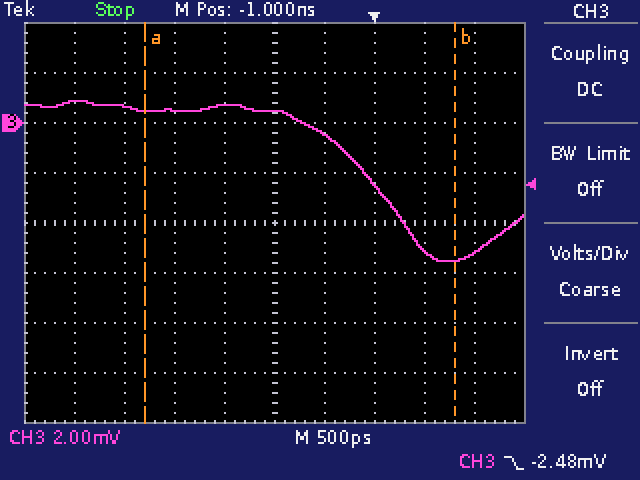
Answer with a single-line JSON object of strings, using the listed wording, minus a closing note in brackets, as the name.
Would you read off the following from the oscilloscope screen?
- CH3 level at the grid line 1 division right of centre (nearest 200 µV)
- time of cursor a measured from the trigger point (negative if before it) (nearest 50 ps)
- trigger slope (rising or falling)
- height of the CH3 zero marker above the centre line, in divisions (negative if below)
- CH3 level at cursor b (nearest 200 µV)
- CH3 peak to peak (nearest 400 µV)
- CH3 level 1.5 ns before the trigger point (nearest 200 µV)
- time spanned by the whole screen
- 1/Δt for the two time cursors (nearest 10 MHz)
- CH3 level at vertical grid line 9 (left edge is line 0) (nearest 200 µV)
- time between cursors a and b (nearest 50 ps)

{"CH3 level at the grid line 1 division right of centre": "-400 µV", "time of cursor a measured from the trigger point (negative if before it)": "-2.30 ns", "trigger slope": "falling", "height of the CH3 zero marker above the centre line, in divisions": "+2.0 div", "CH3 level at cursor b": "-5.4 mV", "CH3 peak to peak": "6.4 mV", "CH3 level 1.5 ns before the trigger point": "800 µV", "time spanned by the whole screen": "5 ns", "1/Δt for the two time cursors": "320 MHz", "CH3 level at vertical grid line 9 (left edge is line 0)": "-5.2 mV", "time between cursors a and b": "3.10 ns"}
